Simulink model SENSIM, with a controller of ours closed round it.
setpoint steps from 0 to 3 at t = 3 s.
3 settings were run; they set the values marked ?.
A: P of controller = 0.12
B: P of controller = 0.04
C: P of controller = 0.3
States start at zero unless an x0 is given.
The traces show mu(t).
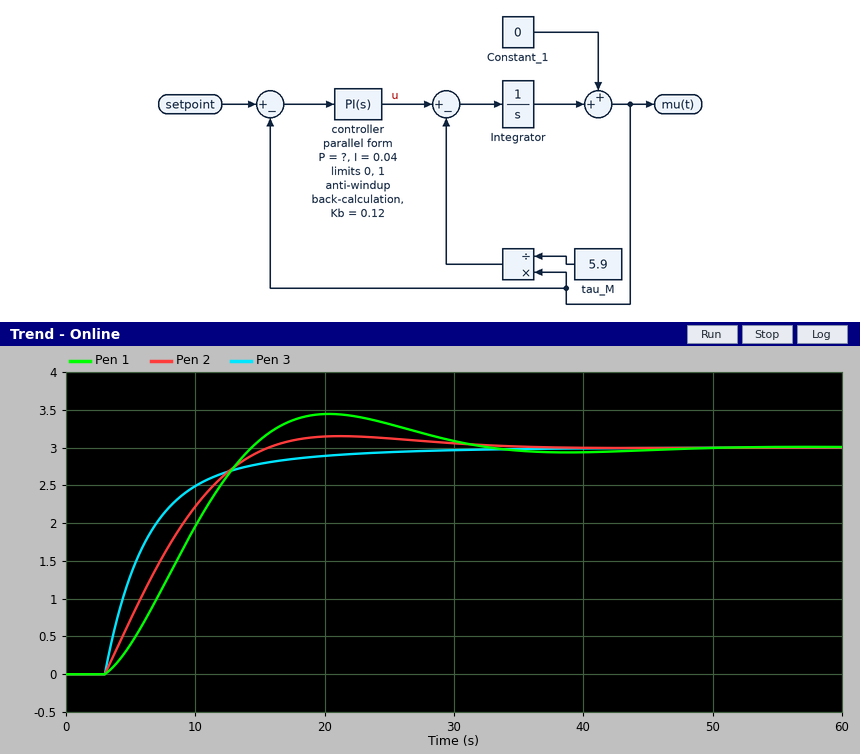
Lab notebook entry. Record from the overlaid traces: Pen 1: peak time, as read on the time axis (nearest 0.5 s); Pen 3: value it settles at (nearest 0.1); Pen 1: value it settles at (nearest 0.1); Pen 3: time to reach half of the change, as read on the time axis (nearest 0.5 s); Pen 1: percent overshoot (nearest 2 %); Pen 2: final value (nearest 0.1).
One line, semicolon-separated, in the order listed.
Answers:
20.5 s; 3.0; 3.0; 5.5 s; 14 %; 3.0
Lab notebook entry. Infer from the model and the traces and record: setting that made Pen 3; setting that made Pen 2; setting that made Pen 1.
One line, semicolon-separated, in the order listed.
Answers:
C; A; B
